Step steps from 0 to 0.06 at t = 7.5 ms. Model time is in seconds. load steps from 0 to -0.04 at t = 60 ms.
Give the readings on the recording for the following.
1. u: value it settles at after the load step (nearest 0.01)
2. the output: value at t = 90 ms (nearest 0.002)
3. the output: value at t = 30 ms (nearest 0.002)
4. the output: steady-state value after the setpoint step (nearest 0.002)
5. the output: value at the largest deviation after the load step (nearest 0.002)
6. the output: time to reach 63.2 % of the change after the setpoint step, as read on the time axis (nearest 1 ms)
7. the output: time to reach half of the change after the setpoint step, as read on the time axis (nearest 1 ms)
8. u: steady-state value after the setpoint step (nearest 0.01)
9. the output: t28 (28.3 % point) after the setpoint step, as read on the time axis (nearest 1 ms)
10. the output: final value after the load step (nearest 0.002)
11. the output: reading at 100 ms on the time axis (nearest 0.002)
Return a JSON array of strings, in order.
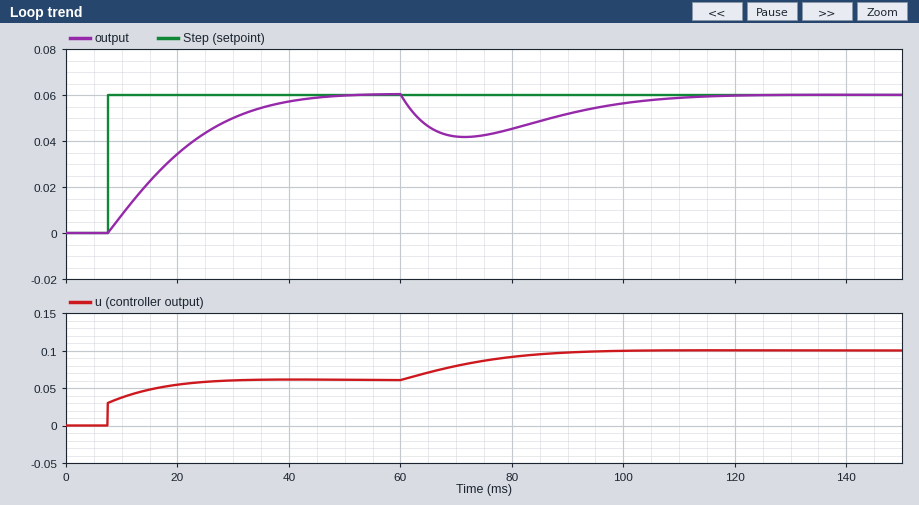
["0.10", "0.052", "0.050", "0.060", "0.042", "22 ms", "18 ms", "0.06", "13 ms", "0.060", "0.056"]
